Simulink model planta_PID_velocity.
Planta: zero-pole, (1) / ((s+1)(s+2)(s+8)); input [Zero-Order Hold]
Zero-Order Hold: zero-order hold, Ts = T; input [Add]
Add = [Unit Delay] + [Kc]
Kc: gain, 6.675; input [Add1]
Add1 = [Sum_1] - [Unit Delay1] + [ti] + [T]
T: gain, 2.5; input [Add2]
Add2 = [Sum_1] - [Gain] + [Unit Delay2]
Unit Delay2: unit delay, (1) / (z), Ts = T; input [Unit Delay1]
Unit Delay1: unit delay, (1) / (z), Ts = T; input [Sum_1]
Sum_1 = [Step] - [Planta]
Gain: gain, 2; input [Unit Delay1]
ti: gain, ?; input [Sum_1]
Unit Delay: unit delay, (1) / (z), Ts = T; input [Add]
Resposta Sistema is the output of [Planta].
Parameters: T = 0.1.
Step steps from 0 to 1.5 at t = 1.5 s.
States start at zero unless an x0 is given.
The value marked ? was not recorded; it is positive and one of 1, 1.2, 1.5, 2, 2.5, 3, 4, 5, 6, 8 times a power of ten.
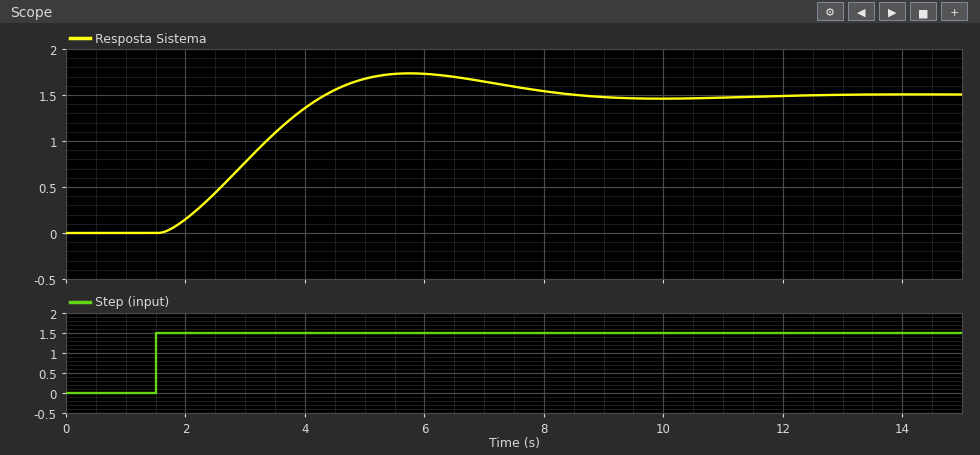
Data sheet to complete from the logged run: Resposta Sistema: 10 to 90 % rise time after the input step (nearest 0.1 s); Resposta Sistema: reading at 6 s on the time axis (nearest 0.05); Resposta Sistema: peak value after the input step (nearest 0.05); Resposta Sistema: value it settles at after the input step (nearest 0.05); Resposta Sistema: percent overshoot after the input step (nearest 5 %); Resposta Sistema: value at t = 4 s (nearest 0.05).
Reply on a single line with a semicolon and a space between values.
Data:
2.0 s; 1.75; 1.75; 1.50; 15 %; 1.35
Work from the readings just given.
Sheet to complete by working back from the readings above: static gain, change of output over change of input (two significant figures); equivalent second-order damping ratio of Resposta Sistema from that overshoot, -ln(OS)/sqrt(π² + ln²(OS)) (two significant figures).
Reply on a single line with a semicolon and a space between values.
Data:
1.0; 0.52
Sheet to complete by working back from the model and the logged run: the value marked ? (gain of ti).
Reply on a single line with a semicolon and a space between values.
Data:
0.2
